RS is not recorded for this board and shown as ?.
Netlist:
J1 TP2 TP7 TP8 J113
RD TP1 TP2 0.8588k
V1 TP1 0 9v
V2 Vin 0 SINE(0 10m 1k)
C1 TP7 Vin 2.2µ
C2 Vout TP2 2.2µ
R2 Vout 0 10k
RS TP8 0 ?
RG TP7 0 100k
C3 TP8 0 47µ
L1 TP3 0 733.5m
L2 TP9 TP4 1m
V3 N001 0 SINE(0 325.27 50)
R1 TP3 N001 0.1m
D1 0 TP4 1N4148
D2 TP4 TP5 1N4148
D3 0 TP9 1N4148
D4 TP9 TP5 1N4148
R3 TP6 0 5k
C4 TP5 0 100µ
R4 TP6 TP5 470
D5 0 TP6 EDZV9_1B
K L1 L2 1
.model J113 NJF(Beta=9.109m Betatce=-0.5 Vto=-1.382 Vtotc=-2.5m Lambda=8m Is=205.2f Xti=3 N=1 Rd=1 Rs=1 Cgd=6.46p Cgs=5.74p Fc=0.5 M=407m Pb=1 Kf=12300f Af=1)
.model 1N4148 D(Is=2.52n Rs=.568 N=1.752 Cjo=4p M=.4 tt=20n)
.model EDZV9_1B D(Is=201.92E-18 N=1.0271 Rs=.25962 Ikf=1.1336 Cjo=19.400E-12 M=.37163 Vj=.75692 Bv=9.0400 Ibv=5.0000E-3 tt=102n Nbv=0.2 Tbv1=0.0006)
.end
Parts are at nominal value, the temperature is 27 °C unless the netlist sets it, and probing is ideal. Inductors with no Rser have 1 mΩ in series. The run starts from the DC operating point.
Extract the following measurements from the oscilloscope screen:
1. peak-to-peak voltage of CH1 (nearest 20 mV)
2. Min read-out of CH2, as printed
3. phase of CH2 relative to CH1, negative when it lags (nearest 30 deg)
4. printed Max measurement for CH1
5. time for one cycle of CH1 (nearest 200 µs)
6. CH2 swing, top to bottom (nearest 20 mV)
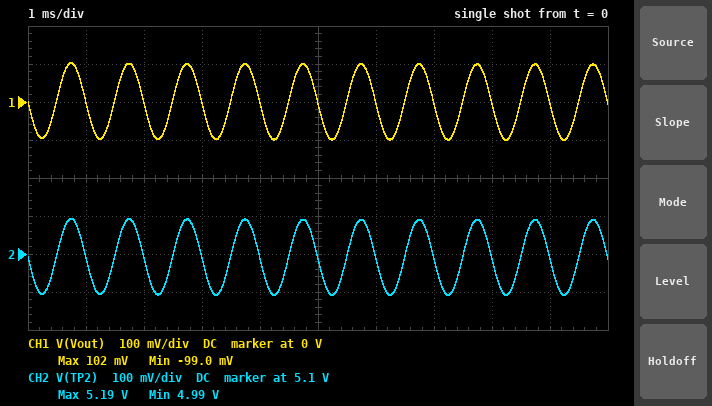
200 mV
4.99 V
0 deg
102 mV
1.0 ms
200 mV
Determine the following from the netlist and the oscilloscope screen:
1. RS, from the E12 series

150 Ω
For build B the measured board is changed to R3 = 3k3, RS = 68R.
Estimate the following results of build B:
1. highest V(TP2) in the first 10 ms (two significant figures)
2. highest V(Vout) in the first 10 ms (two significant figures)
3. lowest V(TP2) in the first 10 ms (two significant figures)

2.9 V
130 mV
2.7 V
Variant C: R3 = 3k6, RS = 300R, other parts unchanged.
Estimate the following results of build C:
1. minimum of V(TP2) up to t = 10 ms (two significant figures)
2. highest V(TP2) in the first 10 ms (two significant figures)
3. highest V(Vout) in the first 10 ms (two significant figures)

6.5 V
6.7 V
81 mV
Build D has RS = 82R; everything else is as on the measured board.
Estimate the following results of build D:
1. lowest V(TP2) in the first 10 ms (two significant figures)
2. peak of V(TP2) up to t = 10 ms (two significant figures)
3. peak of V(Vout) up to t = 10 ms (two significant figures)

3.3 V
3.5 V
120 mV
